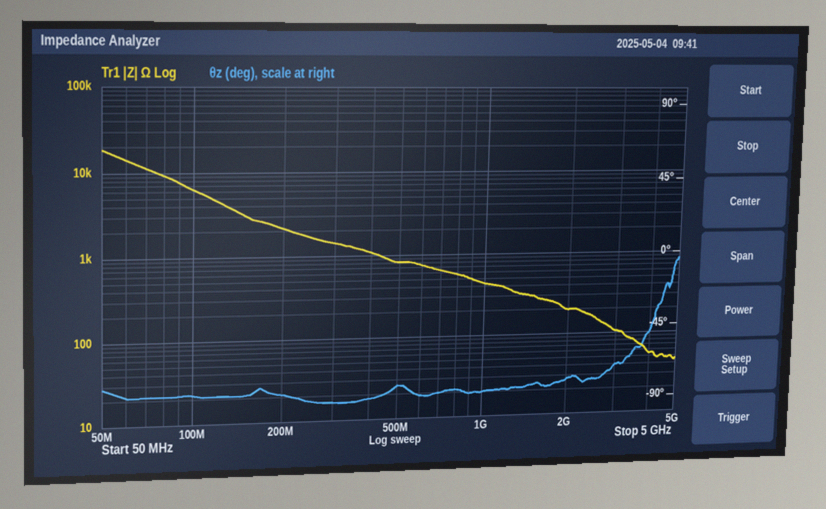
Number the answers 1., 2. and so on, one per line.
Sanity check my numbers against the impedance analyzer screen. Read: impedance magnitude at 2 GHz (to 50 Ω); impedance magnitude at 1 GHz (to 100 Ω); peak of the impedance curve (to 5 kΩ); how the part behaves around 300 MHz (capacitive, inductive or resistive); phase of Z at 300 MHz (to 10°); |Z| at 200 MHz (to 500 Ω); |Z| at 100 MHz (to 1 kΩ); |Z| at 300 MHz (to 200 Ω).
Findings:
1. 200 Ω
2. 400 Ω
3. 20 kΩ
4. capacitive
5. -90°
6. 2.0 kΩ
7. 6 kΩ
8. 1.4 kΩ
